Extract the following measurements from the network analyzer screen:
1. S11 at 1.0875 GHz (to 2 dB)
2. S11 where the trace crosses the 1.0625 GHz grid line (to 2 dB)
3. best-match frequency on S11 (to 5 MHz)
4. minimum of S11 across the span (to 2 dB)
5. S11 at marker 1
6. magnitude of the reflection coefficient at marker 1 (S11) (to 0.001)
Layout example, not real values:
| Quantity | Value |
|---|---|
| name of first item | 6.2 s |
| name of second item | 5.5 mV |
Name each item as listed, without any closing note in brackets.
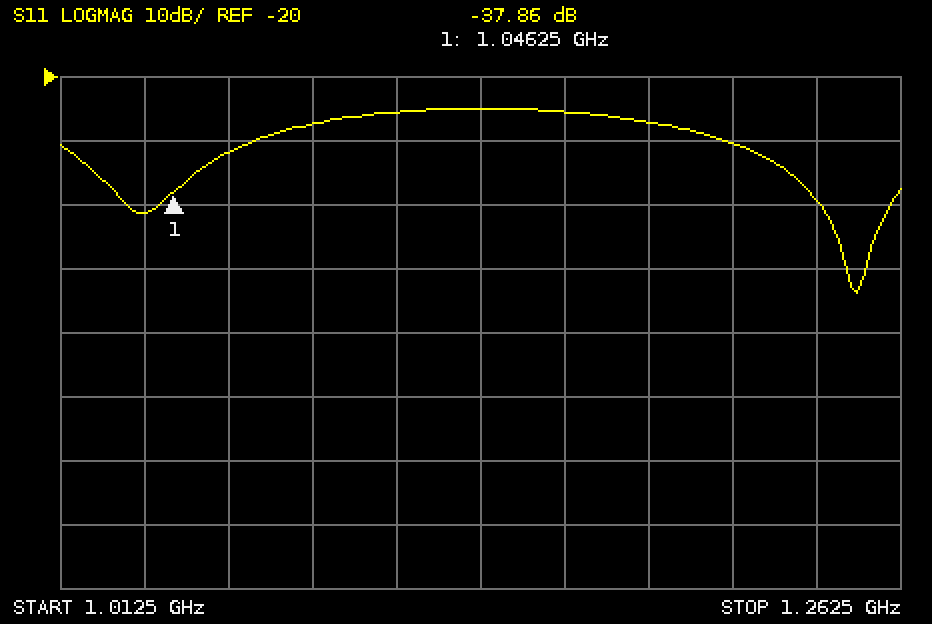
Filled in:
| Quantity | Value |
|---|---|
| S11 at 1.0875 GHz | -28 dB |
| S11 where the trace crosses the 1.0625 GHz grid line | -32 dB |
| best-match frequency on S11 | 1.250 GHz |
| minimum of S11 across the span | -54 dB |
| S11 at marker 1 | -37.86 dB |
| magnitude of the reflection coefficient at marker 1 (S11) | 0.013 |
